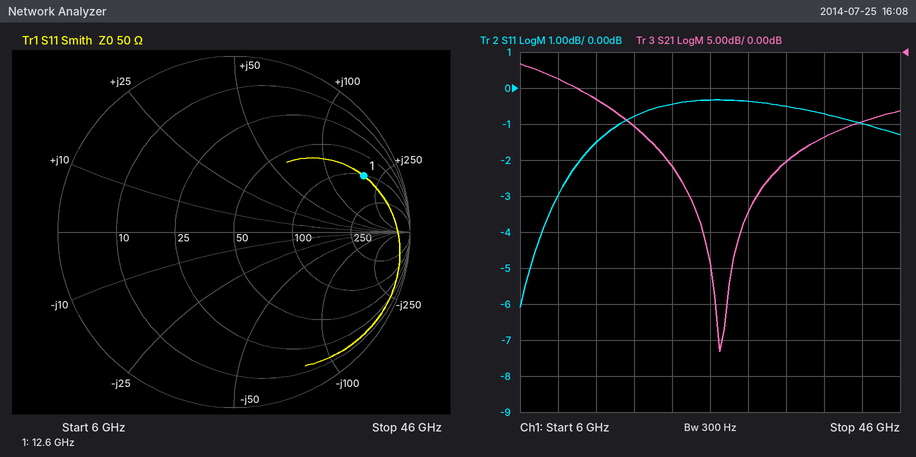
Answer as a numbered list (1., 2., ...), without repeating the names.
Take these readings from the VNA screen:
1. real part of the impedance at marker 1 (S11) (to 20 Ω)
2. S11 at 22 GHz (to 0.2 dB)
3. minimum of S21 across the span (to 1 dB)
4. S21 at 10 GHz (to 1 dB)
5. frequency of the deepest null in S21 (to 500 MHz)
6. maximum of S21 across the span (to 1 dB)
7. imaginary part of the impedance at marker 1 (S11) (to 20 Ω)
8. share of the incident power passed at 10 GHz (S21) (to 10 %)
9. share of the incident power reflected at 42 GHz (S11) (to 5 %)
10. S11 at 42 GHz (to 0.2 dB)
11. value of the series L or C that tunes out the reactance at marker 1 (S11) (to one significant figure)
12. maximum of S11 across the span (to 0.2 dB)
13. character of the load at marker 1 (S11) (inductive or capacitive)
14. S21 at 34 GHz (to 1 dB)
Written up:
1. 100 Ω
2. -0.4 dB
3. -42 dB
4. -4 dB
5. 27.0 GHz
6. -2 dB
7. +180 Ω
8. 40 %
9. 80 %
10. -1.0 dB
11. 70 fF
12. -0.4 dB
13. inductive
14. -15 dB
